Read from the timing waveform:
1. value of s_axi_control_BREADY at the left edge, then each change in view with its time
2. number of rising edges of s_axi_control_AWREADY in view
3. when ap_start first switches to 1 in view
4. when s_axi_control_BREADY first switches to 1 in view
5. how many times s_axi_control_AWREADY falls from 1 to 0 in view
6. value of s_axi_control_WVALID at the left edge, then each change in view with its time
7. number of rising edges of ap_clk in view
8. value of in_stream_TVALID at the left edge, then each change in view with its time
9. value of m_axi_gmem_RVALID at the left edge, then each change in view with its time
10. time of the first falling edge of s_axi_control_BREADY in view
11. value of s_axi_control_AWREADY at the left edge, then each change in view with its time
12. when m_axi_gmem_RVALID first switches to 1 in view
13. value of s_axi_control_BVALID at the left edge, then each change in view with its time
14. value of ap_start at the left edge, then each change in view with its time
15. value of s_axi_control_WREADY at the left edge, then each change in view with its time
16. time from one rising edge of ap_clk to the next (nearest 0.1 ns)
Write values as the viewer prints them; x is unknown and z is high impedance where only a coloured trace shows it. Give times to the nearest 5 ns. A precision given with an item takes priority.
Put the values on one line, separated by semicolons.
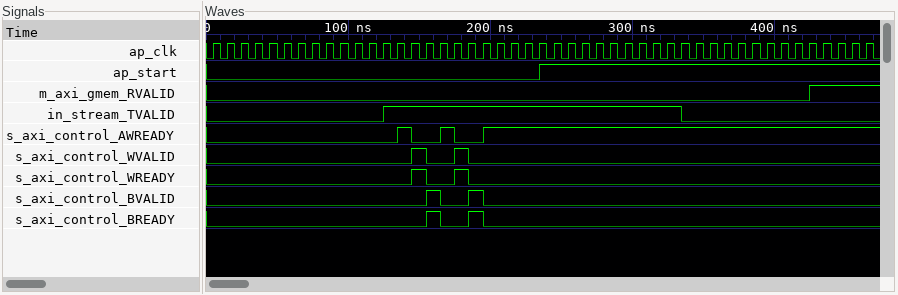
0, 1 at 155 ns, 0 at 165 ns, 1 at 185 ns, 0 at 195 ns; 3; 235 ns; 155 ns; 2; 0, 1 at 145 ns, 0 at 155 ns, 1 at 175 ns, 0 at 185 ns; 47; 0, 1 at 125 ns, 0 at 335 ns; 0, 1 at 425 ns; 165 ns; 0, 1 at 135 ns, 0 at 145 ns, 1 at 165 ns, 0 at 175 ns, 1 at 195 ns; 425 ns; 0, 1 at 155 ns, 0 at 165 ns, 1 at 185 ns, 0 at 195 ns; 0, 1 at 235 ns; 0, 1 at 145 ns, 0 at 155 ns, 1 at 175 ns, 0 at 185 ns; 10 ns
